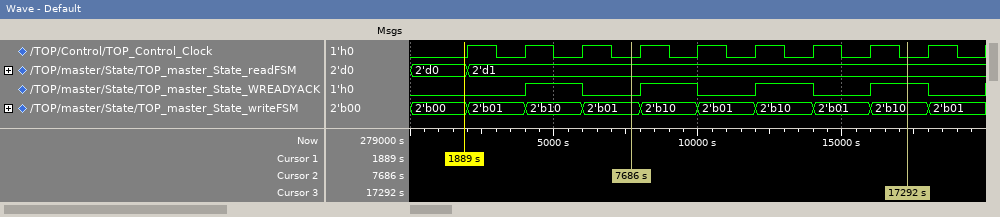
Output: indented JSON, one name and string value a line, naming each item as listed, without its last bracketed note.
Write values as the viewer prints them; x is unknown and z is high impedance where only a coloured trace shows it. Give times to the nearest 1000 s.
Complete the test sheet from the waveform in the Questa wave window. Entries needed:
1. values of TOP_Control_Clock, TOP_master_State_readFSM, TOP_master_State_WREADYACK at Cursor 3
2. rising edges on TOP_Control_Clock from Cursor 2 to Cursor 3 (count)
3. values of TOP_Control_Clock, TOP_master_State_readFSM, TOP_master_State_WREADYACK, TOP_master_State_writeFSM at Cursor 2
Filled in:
{
  "values of TOP_Control_Clock, TOP_master_State_readFSM, TOP_master_State_WREADYACK at Cursor 3": "TOP_Control_Clock=0, TOP_master_State_readFSM=2'd1, TOP_master_State_WREADYACK=1",
  "rising edges on TOP_Control_Clock from Cursor 2 to Cursor 3": "5",
  "values of TOP_Control_Clock, TOP_master_State_readFSM, TOP_master_State_WREADYACK, TOP_master_State_writeFSM at Cursor 2": "TOP_Control_Clock=0, TOP_master_State_readFSM=2'd1, TOP_master_State_WREADYACK=0, TOP_master_State_writeFSM=2'b01"
}
